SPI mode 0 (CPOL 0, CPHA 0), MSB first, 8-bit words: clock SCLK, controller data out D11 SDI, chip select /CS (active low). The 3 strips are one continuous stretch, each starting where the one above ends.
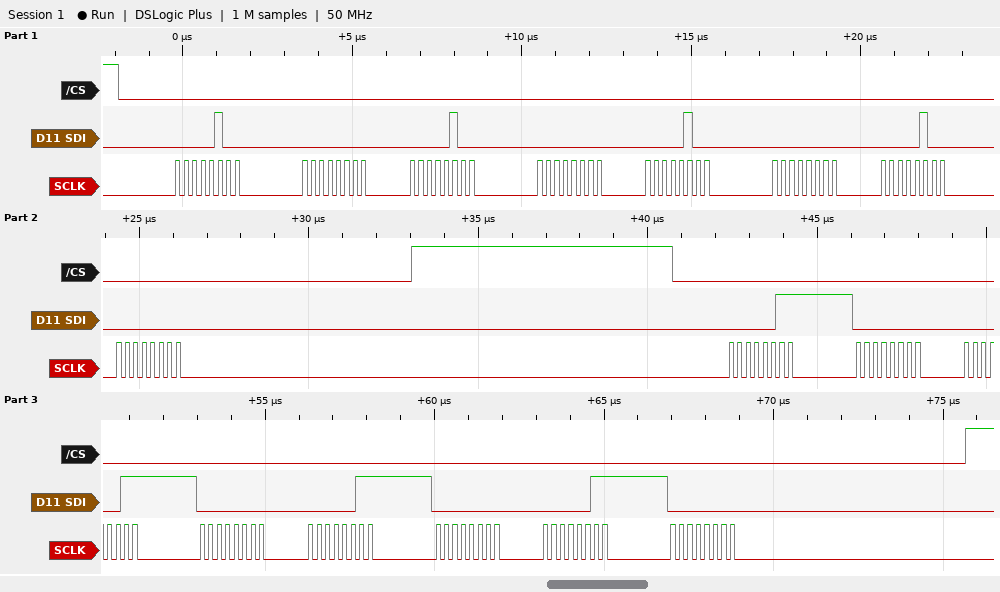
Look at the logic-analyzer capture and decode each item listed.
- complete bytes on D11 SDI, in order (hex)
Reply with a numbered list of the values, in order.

1. 04 00 04 00 04 00 04 00 03 00 03 00 03 00 03 00
